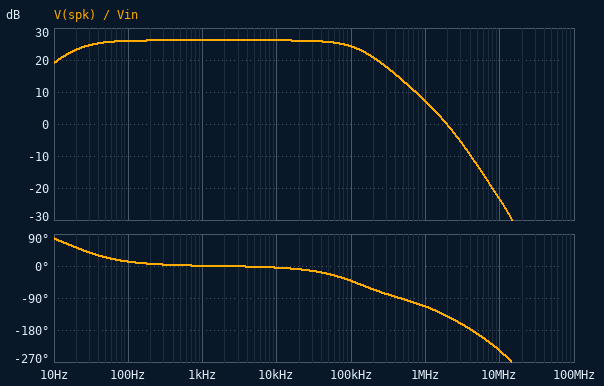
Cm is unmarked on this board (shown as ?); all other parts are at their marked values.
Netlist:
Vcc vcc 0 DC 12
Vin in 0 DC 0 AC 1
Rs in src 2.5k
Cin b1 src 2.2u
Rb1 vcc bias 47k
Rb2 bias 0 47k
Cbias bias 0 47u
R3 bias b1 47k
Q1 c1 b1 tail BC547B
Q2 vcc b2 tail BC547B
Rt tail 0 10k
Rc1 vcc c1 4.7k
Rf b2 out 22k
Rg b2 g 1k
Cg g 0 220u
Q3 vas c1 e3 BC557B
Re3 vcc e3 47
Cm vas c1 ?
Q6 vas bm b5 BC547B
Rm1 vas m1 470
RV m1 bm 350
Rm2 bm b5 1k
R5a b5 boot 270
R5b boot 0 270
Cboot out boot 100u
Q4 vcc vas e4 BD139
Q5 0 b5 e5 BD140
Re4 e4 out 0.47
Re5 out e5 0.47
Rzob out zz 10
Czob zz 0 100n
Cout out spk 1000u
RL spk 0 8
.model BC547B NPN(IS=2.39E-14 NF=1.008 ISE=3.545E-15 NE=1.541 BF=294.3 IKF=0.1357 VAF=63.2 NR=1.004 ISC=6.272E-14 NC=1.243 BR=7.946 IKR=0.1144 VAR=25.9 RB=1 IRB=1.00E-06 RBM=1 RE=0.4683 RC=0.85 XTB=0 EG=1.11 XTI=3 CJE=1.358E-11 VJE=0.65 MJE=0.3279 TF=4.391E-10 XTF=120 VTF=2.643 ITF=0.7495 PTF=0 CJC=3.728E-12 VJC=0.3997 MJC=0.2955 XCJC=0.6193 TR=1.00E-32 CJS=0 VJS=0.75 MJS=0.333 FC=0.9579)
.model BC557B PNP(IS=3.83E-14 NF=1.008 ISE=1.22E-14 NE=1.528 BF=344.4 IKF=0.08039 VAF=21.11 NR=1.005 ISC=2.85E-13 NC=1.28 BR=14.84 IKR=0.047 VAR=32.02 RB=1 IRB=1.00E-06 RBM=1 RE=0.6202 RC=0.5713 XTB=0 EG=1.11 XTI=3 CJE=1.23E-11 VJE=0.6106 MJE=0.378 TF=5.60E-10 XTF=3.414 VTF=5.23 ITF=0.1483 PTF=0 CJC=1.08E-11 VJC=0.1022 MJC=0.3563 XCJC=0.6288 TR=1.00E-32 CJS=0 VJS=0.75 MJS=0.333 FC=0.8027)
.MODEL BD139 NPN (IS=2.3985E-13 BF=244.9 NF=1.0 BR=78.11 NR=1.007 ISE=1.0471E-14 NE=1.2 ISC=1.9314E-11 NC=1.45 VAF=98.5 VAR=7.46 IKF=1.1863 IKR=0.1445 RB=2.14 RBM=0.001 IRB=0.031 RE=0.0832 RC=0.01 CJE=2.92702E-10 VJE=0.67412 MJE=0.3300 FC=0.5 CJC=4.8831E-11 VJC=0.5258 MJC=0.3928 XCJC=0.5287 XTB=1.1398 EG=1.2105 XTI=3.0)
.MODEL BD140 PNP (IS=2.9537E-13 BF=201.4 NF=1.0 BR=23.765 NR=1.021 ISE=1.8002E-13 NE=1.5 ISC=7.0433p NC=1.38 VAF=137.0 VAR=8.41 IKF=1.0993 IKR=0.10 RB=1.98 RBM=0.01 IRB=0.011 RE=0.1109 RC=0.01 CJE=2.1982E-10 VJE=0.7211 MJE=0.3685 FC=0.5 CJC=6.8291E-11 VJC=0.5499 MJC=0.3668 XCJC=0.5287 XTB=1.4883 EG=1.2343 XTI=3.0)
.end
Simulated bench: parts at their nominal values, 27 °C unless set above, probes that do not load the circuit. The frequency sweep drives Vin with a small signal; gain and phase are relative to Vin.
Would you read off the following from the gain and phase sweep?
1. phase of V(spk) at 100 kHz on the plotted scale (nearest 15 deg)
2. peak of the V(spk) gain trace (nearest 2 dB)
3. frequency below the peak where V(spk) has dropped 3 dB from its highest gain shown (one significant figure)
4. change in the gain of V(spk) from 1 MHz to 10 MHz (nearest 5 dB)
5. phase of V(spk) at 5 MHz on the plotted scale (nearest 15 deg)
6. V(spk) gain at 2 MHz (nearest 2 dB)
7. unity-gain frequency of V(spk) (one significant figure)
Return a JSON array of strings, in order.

["-45 deg", "26 dB", "20 Hz", "-30 dB", "-195 deg", "0 dB", "2 MHz"]
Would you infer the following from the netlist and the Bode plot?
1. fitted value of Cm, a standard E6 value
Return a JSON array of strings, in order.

["220 pF"]
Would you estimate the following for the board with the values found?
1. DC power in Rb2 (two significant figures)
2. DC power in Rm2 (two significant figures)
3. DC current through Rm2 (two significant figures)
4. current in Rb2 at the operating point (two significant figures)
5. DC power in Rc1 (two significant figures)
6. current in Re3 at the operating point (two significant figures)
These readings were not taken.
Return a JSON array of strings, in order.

["760 µW", "490 µW", "700 µA", "130 µA", "280 µW", "9.8 mA"]
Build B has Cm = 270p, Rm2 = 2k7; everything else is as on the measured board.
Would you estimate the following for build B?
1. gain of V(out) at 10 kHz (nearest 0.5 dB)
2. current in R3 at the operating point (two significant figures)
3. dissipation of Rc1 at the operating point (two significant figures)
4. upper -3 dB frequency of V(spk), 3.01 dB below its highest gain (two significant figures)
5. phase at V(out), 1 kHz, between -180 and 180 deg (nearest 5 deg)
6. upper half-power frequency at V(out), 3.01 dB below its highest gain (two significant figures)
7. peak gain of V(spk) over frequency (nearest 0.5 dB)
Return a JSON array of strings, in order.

["9.5 dB", "910 nA", "290 µW", "26 kHz", "-5 deg", "7.1 Hz", "10.0 dB"]
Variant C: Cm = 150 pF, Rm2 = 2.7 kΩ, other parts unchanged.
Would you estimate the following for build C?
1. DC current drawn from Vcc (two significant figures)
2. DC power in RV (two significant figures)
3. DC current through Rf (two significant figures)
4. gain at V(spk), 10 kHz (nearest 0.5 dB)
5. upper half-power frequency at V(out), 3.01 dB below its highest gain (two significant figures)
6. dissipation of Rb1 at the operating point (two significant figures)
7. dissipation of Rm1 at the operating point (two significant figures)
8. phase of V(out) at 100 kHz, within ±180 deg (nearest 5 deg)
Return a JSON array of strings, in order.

["11 mA", "31 µW", "820 nA", "10.0 dB", "7.1 Hz", "770 µW", "42 µW", "-80 deg"]
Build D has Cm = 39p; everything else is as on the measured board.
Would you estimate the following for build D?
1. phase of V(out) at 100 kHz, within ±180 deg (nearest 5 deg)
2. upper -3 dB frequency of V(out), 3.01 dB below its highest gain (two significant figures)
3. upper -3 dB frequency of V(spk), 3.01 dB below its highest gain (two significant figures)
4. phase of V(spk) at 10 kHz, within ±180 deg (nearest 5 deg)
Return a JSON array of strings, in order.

["-10 deg", "690 kHz", "700 kHz", "0 deg"]
